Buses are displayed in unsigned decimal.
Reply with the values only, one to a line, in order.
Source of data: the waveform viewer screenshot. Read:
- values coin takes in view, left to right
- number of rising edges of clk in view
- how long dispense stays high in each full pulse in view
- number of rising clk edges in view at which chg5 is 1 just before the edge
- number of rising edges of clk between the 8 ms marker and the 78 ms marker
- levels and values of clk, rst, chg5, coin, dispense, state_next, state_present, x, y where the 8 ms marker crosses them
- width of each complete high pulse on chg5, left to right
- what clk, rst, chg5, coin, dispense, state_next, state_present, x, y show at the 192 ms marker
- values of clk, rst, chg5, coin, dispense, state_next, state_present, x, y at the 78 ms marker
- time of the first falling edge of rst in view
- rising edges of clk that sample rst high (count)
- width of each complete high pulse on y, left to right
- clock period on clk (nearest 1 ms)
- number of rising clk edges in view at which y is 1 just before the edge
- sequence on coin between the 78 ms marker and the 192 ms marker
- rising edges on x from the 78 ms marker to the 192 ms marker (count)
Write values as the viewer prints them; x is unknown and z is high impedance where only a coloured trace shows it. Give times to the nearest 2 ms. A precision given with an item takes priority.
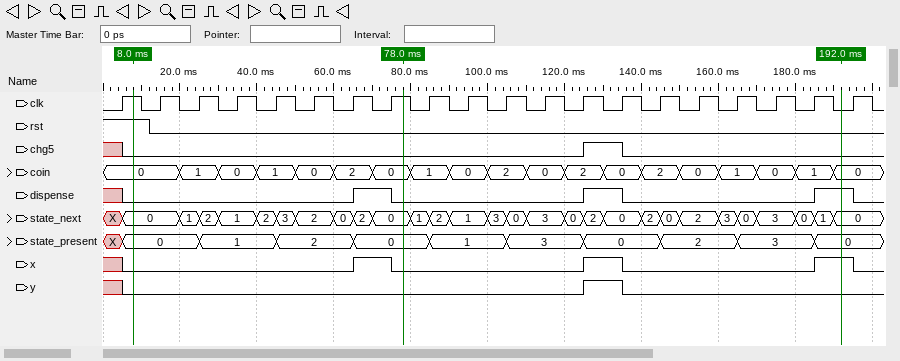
0, 1, 0, 1, 0, 2, 0, 1, 0, 2, 0, 2, 0, 2, 0, 1, 0, 1, 0
20
10 ms, 10 ms, 10 ms
1
7
clk=1, rst=1, chg5=0, coin=0, dispense=0, state_next=0, state_present=0, x=0, y=0
10 ms
clk=0, rst=0, chg5=0, coin=0, dispense=1, state_next=0, state_present=0, x=1, y=0
clk=1, rst=0, chg5=0, coin=0, dispense=0, state_next=0, state_present=0, x=0, y=0
12 ms
1
10 ms
10 ms
1
0, 1, 0, 2, 0, 2, 0, 2, 0, 1, 0, 1, 0
2
